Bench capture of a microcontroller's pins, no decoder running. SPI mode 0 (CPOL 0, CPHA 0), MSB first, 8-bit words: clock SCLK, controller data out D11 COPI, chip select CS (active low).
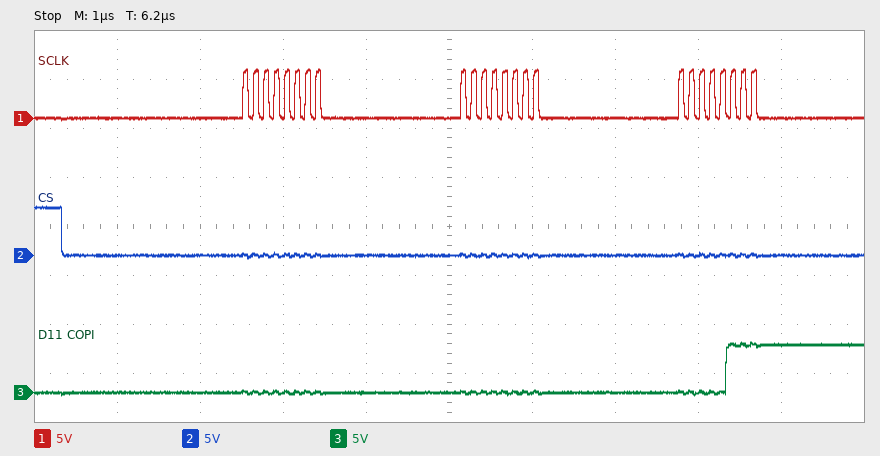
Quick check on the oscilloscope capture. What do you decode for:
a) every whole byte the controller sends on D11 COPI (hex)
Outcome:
00 00 07
